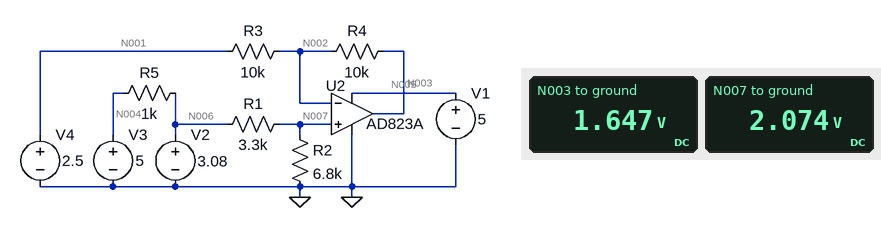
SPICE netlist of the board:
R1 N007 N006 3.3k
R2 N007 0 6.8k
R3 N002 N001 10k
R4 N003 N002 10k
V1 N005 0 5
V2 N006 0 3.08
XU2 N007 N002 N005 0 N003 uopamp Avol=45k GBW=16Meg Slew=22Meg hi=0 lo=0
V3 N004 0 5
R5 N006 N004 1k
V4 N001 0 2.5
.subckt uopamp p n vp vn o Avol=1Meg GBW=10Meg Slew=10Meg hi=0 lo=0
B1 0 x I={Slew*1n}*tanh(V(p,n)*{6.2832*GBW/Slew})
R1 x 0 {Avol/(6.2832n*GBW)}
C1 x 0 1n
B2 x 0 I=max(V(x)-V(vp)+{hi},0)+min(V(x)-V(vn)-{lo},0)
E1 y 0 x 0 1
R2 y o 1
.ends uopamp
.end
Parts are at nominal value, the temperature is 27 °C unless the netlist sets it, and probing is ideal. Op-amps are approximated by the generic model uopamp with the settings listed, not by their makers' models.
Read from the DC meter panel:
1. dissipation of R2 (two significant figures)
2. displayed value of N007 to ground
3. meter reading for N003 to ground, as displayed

630 µW
2.074 V
1.647 V
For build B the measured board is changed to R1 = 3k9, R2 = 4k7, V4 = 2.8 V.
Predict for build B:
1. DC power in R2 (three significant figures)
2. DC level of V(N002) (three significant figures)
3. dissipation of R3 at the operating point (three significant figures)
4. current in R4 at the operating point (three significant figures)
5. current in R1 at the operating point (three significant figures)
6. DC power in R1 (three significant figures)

603 µW
1.68 V
125 µW
112 µA
358 µA
500 µW
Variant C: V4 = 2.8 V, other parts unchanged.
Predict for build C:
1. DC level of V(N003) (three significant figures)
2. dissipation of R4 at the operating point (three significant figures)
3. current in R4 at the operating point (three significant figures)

1.35 V
52.8 µW
72.6 µA
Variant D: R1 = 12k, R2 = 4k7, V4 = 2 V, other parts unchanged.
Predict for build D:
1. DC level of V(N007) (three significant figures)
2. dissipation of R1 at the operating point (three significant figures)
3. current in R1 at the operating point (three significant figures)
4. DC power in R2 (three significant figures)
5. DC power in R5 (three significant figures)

867 mV
408 µW
184 µA
160 µW
3.69 mW
